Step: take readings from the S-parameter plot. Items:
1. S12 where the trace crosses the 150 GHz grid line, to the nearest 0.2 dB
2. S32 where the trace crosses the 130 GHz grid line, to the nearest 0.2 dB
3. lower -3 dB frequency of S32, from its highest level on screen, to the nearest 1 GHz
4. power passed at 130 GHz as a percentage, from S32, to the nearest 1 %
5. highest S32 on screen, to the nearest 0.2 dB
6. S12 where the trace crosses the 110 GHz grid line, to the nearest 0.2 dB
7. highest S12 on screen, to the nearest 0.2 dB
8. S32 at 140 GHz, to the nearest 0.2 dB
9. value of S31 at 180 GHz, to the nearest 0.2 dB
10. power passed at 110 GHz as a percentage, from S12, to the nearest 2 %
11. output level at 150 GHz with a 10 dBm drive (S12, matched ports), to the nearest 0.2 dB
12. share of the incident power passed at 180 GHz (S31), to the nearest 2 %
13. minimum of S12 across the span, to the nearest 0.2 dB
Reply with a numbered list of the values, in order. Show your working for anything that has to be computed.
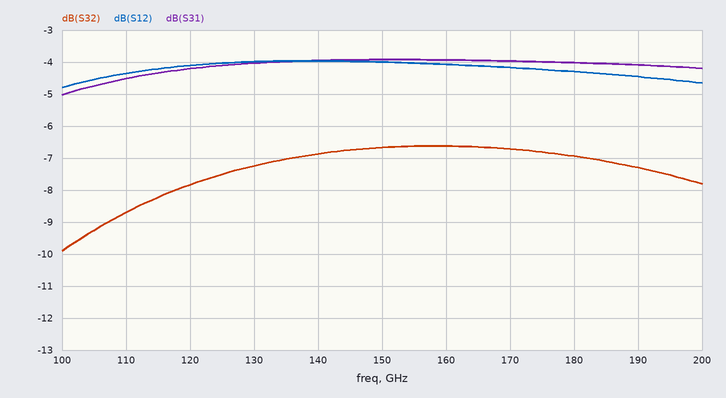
1. -4.0 dB
2. -7.2 dB
3. 102 GHz
4. 10^(-7.2/10) ≈ 19 %
5. -6.6 dB
6. -4.4 dB
7. -4.0 dB
8. -6.8 dB
9. -4.0 dB
10. 10^(-4.4/10) ≈ 36 %
11. 10 dBm + (-4.0 dB) = 6.0 dBm
12. 10^(-4/10) ≈ 40 %
13. -4.8 dB
